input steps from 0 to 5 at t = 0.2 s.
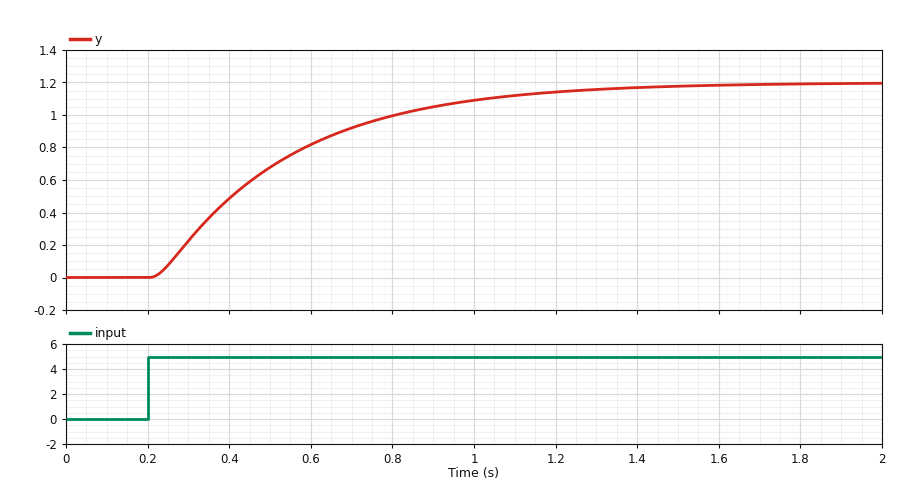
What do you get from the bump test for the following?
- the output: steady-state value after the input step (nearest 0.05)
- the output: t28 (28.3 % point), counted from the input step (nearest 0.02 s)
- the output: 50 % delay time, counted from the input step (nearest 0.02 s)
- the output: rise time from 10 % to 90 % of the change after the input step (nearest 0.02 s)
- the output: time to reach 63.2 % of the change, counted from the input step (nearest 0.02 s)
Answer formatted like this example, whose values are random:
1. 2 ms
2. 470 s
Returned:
1. 1.20
2. 0.14 s
3. 0.26 s
4. 0.70 s
5. 0.36 s
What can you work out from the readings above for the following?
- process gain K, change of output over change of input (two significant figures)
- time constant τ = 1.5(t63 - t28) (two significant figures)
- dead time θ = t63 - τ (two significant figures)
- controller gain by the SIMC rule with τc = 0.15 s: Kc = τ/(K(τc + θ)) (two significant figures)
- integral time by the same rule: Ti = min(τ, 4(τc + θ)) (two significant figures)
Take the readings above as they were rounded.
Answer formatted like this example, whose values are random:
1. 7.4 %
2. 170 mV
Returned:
1. 0.24
2. 0.33 s
3. 0.030 s
4. 7.6
5. 0.33 s
